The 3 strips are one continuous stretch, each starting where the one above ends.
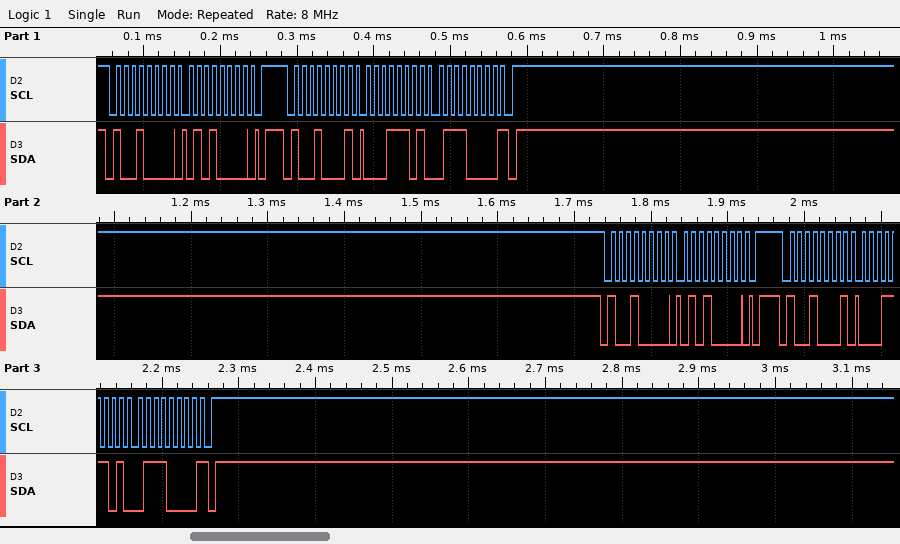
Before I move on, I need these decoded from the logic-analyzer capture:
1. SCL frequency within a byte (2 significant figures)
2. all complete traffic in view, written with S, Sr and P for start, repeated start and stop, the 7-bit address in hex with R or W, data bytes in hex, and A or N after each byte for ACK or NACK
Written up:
100 kHz
S 48W A 50 A P S 48R A 1D A 70 N P S 48W A 50 A P S 48R A 1D A 70 N P
